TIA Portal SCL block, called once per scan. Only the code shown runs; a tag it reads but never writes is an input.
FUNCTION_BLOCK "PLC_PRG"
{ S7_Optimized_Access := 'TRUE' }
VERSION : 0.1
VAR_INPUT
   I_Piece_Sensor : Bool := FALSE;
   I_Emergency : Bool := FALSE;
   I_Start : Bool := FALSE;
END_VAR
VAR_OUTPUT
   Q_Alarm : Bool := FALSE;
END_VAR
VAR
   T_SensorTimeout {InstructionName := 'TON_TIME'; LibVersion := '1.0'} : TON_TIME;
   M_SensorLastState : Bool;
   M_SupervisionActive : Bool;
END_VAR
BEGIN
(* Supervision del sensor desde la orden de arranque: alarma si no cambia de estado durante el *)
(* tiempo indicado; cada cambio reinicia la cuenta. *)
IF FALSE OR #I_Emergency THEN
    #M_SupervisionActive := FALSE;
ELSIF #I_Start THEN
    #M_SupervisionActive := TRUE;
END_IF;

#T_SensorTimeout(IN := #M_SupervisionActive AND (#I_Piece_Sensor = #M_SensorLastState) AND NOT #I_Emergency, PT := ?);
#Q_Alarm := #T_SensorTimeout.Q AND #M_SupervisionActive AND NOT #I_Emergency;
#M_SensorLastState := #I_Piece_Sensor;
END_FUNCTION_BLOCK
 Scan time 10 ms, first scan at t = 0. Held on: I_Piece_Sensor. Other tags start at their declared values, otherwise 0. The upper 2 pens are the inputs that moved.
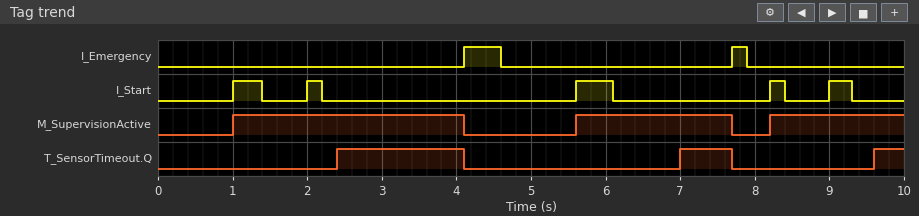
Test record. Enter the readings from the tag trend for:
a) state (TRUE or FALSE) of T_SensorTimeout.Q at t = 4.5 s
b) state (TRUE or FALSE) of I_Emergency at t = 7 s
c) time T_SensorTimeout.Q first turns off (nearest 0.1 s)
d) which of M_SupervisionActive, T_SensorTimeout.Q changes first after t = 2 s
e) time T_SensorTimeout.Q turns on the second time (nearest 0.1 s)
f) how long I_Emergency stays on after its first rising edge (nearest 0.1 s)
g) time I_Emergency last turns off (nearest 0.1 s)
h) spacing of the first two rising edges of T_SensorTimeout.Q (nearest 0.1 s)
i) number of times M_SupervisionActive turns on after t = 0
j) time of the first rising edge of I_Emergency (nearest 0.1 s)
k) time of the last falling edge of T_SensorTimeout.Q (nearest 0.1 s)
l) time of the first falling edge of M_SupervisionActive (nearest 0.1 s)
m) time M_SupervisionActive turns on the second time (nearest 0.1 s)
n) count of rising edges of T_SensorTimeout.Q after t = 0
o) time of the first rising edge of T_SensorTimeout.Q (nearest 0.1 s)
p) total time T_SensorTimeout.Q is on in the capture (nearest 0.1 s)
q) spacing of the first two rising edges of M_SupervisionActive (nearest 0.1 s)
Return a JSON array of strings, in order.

["FALSE", "FALSE", "4.1 s", "T_SensorTimeout.Q", "7.0 s", "0.5 s", "7.9 s", "4.6 s", "3", "4.1 s", "7.7 s", "4.1 s", "5.6 s", "3", "2.4 s", "2.8 s", "4.6 s"]
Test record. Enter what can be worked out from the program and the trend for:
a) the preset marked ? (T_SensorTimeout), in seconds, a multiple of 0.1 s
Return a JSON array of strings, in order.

["1.4 s"]
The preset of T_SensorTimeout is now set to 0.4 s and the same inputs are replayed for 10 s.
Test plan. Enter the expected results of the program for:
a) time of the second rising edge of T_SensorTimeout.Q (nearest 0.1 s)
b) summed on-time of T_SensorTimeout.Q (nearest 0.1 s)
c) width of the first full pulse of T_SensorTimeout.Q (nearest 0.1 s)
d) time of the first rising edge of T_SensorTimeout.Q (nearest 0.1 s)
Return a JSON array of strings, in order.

["6.0 s", "5.8 s", "2.7 s", "1.4 s"]
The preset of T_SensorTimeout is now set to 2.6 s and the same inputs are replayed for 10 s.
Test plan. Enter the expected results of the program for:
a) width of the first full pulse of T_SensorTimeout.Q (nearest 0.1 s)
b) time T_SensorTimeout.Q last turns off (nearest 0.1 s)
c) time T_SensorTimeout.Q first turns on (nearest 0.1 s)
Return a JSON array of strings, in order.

["0.5 s", "4.1 s", "3.6 s"]
